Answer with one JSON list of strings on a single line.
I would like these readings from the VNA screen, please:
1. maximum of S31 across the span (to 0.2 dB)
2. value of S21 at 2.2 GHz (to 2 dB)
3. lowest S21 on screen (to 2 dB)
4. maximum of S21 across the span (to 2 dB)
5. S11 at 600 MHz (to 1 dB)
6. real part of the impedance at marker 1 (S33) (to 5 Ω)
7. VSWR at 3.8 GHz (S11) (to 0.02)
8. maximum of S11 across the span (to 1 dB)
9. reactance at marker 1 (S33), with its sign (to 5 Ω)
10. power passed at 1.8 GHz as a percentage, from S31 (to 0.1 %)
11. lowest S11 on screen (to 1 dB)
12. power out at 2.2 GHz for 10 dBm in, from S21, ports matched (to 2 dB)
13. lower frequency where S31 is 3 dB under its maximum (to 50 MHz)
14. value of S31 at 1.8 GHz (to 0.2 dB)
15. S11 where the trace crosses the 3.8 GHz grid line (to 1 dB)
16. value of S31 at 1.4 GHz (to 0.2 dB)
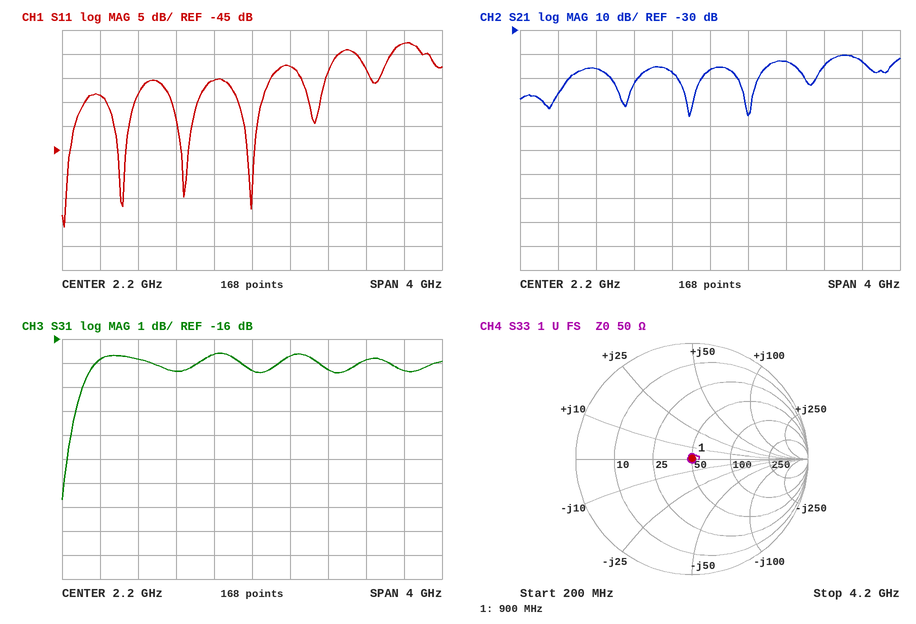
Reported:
["-16.6 dB", "-46 dB", "-66 dB", "-40 dB", "-34 dB", "50 Ω", "1.16", "-23 dB", "0 Ω", "2.2 %", "-61 dB", "-36 dBm", "300 MHz", "-16.6 dB", "-23 dB", "-17.4 dB"]
